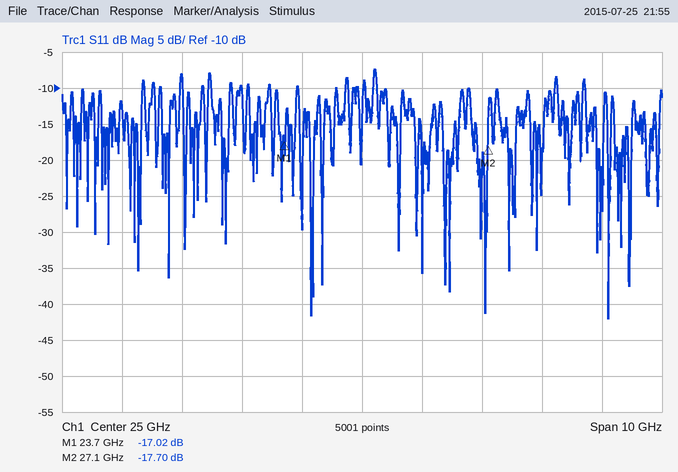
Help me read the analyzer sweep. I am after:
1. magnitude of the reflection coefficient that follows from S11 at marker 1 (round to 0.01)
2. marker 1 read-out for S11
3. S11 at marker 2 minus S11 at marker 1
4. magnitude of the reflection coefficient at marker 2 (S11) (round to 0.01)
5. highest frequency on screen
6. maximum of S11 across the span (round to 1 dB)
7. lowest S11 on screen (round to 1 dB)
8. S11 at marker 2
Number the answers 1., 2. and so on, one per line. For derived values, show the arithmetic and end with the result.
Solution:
1. 10^(-17.02/20) ≈ 0.14
2. -17.02 dB
3. -17.7 − (-17.02) = -0.68 dB
4. 10^(-17.7/20) ≈ 0.13
5. 30 GHz
6. -7 dB
7. -42 dB
8. -17.70 dB
